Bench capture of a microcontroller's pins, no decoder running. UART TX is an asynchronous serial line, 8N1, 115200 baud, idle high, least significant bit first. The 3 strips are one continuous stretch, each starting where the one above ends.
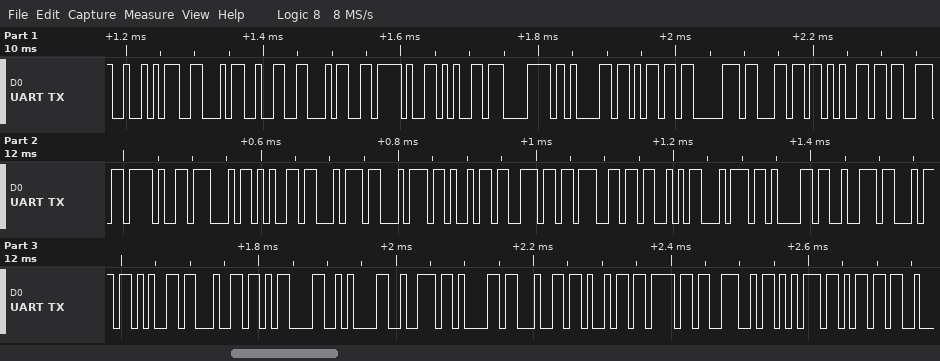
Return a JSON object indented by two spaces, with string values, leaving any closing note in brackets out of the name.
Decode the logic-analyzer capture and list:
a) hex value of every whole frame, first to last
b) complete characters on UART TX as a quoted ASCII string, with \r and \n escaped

{
  "hex value of every whole frame, first to last": "52 46 32 34 2F 65 78 61 6D 70 6C 65 73 2F 47 65 74 74 69 6E 67 53 74 61 72 74 65 64 0D 0A 72 61 64 69 6F 4E 75 6D",
  "complete characters on UART TX as a quoted ASCII string, with \\r and \\n escaped": "\"RF24/examples/GettingStarted\\r\\nradioNum\""
}
